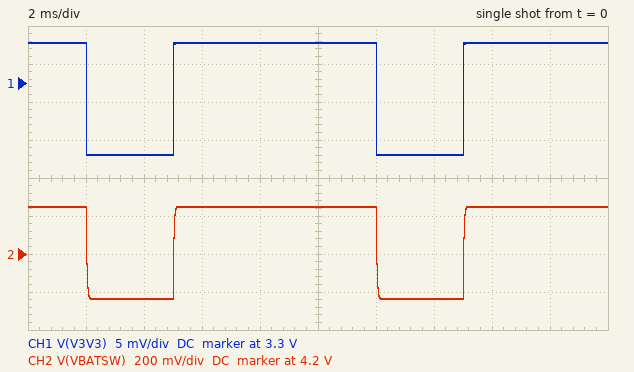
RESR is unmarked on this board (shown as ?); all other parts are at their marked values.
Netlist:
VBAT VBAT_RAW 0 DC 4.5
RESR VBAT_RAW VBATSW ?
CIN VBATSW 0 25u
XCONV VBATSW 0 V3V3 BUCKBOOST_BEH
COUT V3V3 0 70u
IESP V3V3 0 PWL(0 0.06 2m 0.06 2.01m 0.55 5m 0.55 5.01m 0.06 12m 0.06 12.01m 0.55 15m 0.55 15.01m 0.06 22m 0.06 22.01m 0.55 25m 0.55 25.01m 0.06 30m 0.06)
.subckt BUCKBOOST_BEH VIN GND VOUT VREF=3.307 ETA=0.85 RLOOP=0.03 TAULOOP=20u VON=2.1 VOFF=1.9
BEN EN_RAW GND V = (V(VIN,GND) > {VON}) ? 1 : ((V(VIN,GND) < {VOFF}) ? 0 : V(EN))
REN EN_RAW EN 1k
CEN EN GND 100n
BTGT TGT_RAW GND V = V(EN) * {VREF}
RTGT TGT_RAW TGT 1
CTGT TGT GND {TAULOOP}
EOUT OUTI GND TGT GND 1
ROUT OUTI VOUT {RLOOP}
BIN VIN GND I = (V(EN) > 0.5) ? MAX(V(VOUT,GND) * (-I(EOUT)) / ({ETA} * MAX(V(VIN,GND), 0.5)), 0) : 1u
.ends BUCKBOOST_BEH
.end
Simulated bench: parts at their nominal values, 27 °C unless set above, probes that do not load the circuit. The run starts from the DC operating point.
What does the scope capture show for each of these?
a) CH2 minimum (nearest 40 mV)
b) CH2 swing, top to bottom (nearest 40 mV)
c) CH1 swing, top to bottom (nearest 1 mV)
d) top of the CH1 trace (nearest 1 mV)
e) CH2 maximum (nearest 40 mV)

3.96 V
480 mV
15 mV
3.305 V
4.44 V
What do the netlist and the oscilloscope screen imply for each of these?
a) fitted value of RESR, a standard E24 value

1 Ω
